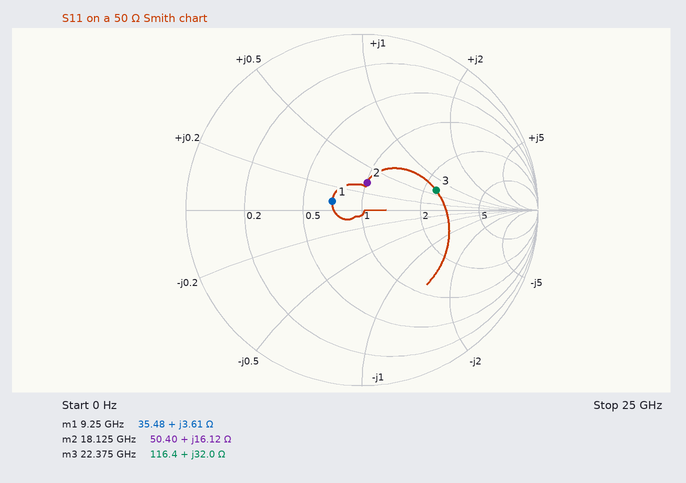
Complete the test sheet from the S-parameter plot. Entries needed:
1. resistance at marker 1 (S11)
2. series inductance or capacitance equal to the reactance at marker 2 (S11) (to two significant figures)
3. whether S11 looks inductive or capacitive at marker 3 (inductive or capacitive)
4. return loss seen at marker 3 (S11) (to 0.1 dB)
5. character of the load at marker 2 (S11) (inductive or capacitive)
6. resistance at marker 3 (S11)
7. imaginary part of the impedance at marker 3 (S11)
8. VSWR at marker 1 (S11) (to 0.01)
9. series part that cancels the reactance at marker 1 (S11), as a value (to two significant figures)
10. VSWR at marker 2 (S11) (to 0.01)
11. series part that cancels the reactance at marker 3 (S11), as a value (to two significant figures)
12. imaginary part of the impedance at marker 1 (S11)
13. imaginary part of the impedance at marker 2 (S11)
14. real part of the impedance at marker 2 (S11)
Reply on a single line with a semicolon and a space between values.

35.48 Ω; 140 pH; inductive; 7.2 dB; inductive; 116.4 Ω; +32.0 Ω; 1.42; 4.8 pF; 1.38; 220 fF; +3.61 Ω; +16.12 Ω; 50.40 Ω
